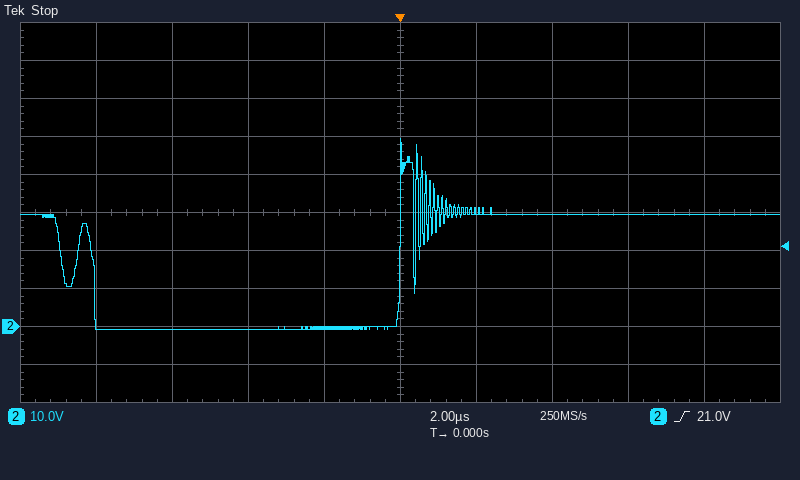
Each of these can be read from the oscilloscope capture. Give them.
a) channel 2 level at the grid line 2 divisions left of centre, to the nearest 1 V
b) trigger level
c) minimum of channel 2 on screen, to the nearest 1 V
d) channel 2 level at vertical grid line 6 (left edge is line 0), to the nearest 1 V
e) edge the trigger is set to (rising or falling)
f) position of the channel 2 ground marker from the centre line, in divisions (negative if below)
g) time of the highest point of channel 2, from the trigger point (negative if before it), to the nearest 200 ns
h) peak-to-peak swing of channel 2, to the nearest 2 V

-1 V
21.0 V
-1 V
30 V
rising
-3.0 div
0.0 µs
50 V
